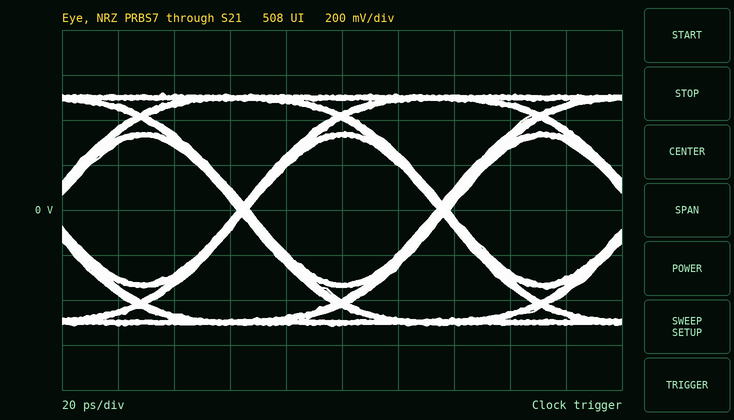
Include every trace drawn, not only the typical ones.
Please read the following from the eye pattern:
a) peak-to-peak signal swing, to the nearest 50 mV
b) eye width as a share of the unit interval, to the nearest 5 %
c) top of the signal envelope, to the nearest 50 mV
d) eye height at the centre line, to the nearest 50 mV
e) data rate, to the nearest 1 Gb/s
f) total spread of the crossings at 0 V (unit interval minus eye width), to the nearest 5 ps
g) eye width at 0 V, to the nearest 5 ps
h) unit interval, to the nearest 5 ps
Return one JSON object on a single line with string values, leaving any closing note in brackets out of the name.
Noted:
{"peak-to-peak signal swing, to the nearest 50 mV": "1.05 V", "eye width as a share of the unit interval, to the nearest 5 %": "95 %", "top of the signal envelope, to the nearest 50 mV": "500 mV", "eye height at the centre line, to the nearest 50 mV": "650 mV", "data rate, to the nearest 1 Gb/s": "14 Gb/s", "total spread of the crossings at 0 V (unit interval minus eye width), to the nearest 5 ps": "5 ps", "eye width at 0 V, to the nearest 5 ps": "65 ps", "unit interval, to the nearest 5 ps": "70 ps"}
